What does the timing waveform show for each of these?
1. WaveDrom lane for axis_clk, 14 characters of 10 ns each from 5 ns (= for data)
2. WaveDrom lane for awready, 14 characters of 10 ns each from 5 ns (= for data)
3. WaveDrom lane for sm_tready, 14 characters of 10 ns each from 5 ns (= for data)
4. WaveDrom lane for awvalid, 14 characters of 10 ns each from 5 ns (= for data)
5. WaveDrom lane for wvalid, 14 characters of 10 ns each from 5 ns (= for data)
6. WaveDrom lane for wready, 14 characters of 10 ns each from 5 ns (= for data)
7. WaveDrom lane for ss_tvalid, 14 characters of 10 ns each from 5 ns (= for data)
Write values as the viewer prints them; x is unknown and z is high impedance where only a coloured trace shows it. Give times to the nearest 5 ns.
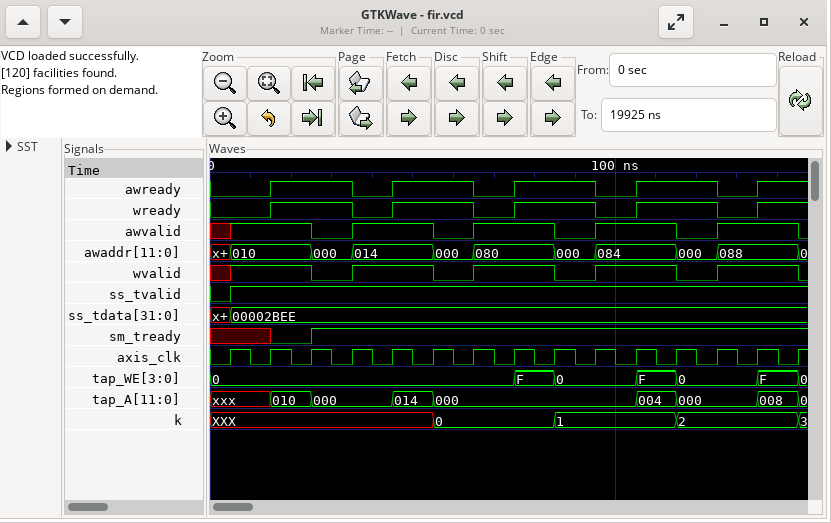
{name: 'axis_clk', wave: 'p.............'}
{name: 'awready', wave: '01.01.01.01.01'}
{name: 'sm_tready', wave: 'x01...........'}
{name: 'awvalid', wave: '1.01.01.01.01.'}
{name: 'wvalid', wave: '1.01.01.01.01.'}
{name: 'wready', wave: '01.01.01.01.01'}
{name: 'ss_tvalid', wave: '1.............'}
